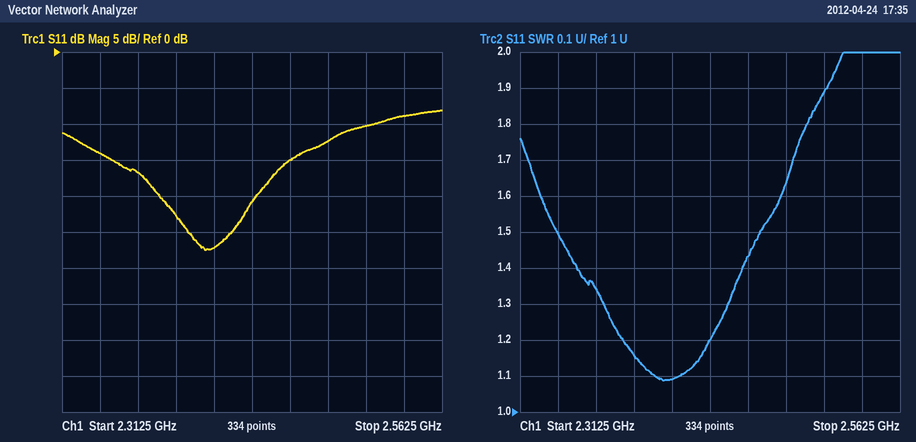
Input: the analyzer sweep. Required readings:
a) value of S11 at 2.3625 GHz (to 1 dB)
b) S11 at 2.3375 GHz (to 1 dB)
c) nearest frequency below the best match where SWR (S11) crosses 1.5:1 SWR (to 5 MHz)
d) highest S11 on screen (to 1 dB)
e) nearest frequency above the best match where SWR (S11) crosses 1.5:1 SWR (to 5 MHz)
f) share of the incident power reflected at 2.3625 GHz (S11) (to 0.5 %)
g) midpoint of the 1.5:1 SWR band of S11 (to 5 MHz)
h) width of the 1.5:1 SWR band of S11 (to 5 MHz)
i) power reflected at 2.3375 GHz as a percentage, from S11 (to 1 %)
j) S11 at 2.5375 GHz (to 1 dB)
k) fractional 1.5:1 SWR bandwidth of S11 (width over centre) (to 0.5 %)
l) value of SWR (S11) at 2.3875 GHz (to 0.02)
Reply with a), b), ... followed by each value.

a) -17 dB
b) -14 dB
c) 2.335 GHz
d) -8 dB
e) 2.470 GHz
f) 2.0 %
g) 2.405 GHz
h) 135 MHz
i) 4 %
j) -9 dB
k) 5.5 %
l) 1.16
